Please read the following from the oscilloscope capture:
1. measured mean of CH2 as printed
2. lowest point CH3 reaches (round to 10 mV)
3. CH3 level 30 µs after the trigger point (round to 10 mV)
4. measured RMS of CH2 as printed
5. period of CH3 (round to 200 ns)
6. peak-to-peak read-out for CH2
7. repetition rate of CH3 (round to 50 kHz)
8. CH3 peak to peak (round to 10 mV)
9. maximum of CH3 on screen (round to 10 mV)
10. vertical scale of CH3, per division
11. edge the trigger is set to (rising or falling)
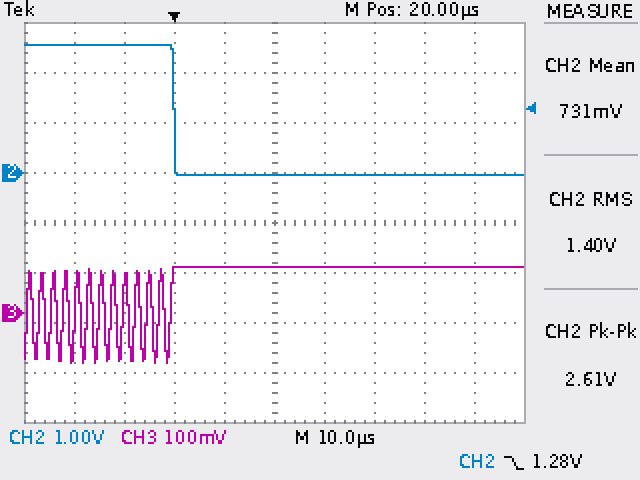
731 mV
-100 mV
90 mV
1.40 V
2.4 µs
2.61 V
400 kHz
190 mV
90 mV
100 mV
falling
